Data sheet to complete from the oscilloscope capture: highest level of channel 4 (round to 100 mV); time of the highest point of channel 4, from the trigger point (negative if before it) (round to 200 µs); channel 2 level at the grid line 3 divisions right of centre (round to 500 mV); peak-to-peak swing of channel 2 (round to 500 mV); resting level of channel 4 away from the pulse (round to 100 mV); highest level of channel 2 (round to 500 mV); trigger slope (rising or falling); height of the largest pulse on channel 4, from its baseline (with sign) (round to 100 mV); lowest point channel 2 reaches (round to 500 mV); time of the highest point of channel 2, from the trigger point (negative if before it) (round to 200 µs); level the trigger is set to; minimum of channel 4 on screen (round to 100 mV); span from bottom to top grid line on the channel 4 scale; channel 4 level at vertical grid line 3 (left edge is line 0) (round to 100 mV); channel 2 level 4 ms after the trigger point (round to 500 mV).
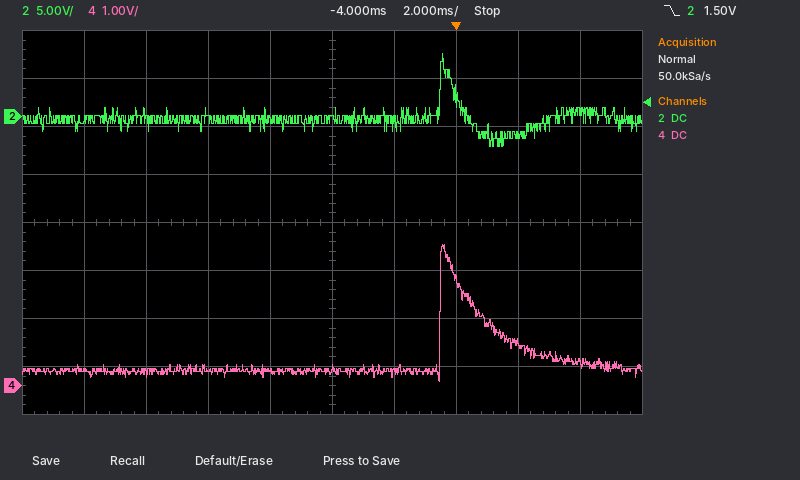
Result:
2.9 V
-400 µs
-2.0 V
9.5 V
300 mV
6.5 V
falling
+2.6 V
-3.0 V
-400 µs
1.50 V
100 mV
8 V
300 mV
500 mV
